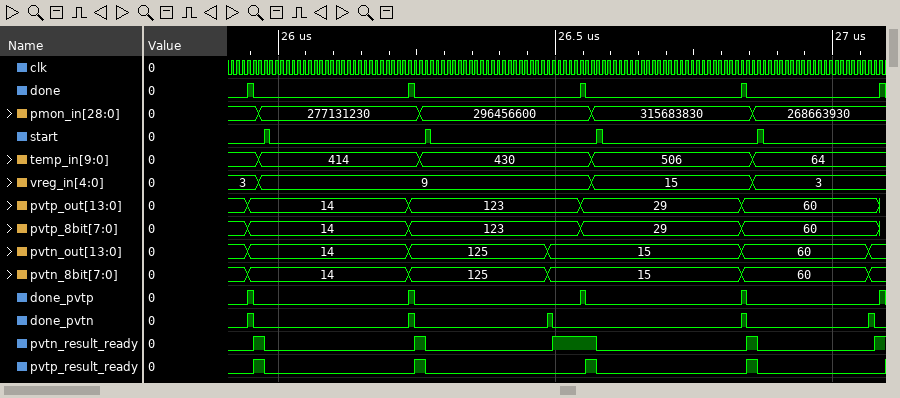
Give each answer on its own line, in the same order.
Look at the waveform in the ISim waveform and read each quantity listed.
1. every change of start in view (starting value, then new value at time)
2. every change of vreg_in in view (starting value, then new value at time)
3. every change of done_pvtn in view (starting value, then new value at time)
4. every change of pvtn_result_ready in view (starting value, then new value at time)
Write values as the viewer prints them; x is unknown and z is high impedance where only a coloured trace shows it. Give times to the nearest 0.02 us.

0, 1 at 25.98 us, 0 at 25.98 us, 1 at 26.26 us, 0 at 26.28 us, 1 at 26.58 us, 0 at 26.58 us, 1 at 26.86 us, 0 at 26.88 us
3, 9 at 25.96 us, 15 at 26.56 us, 3 at 26.86 us
0, 1 at 25.94 us, 0 at 25.96 us, 1 at 26.24 us, 0 at 26.24 us, 1 at 26.48 us, 0 at 26.5 us, 1 at 26.84 us, 0 at 26.84 us, 1 at 27.06 us, 0 at 27.08 us
0, 1 at 25.96 us, 0 at 25.98 us, 1 at 26.24 us, 0 at 26.26 us, 1 at 26.5 us, 0 at 26.58 us, 1 at 26.84 us, 0 at 26.86 us, 1 at 27.08 us
